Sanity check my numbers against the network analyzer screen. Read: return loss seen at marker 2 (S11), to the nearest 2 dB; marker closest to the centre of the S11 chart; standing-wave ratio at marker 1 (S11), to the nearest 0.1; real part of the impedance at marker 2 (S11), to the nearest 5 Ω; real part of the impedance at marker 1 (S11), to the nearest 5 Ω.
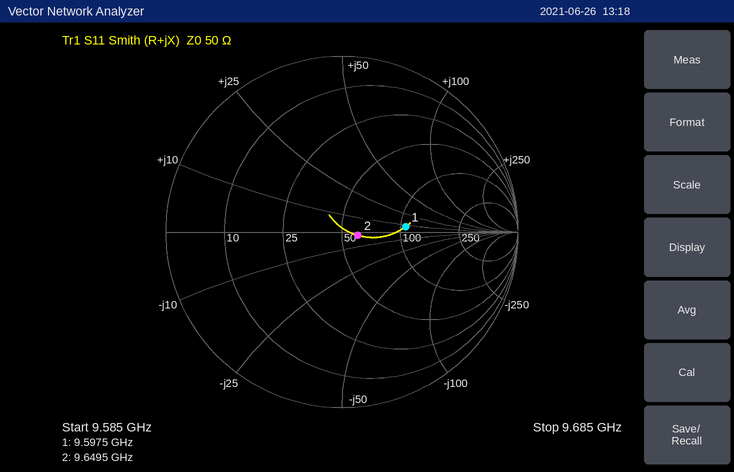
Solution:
20 dB
marker 2
2.1
60 Ω
105 Ω
